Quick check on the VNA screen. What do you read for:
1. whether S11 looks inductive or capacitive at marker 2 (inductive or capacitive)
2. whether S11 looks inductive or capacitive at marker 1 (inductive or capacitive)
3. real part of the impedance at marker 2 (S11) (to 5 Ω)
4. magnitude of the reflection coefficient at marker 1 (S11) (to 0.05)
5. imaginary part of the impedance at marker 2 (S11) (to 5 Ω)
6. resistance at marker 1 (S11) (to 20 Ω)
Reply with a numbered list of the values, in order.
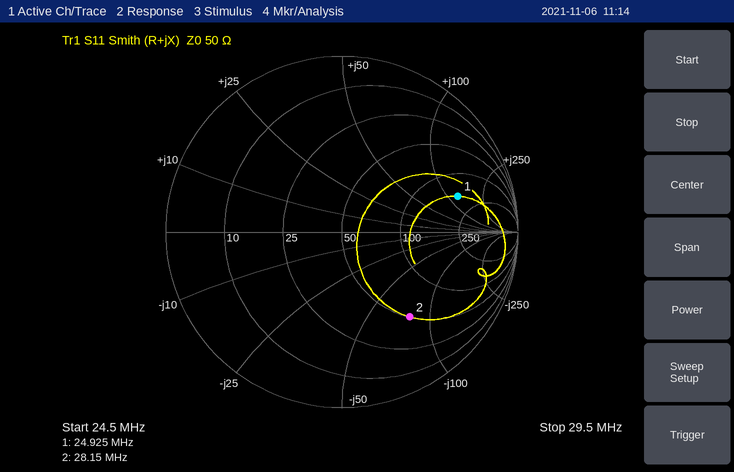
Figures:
1. capacitive
2. inductive
3. 50 Ω
4. 0.70
5. -80 Ω
6. 160 Ω
